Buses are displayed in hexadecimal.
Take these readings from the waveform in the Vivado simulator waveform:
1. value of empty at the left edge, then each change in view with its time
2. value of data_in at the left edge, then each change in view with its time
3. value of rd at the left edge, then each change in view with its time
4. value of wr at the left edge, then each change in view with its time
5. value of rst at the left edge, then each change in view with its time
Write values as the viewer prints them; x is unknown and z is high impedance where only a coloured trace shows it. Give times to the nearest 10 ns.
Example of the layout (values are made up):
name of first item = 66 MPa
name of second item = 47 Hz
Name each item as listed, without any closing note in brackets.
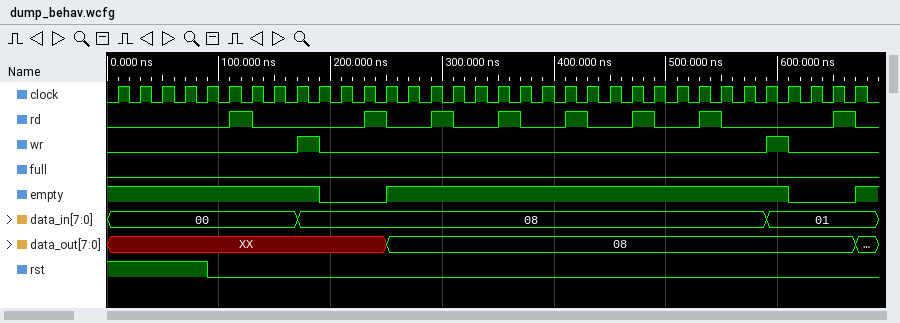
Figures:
value of empty at the left edge, then each change in view with its time = 1, 0 at 190 ns, 1 at 250 ns, 0 at 610 ns, 1 at 670 ns
value of data_in at the left edge, then each change in view with its time = 00, 08 at 170 ns, 01 at 590 ns
value of rd at the left edge, then each change in view with its time = 0, 1 at 110 ns, 0 at 130 ns, 1 at 230 ns, 0 at 250 ns, 1 at 290 ns, 0 at 310 ns, 1 at 350 ns, 0 at 370 ns, 1 at 410 ns, 0 at 430 ns, 1 at 470 ns, 0 at 490 ns, 1 at 530 ns, 0 at 550 ns, 1 at 650 ns, 0 at 670 ns
value of wr at the left edge, then each change in view with its time = 0, 1 at 170 ns, 0 at 190 ns, 1 at 590 ns, 0 at 610 ns
value of rst at the left edge, then each change in view with its time = 1, 0 at 90 ns
